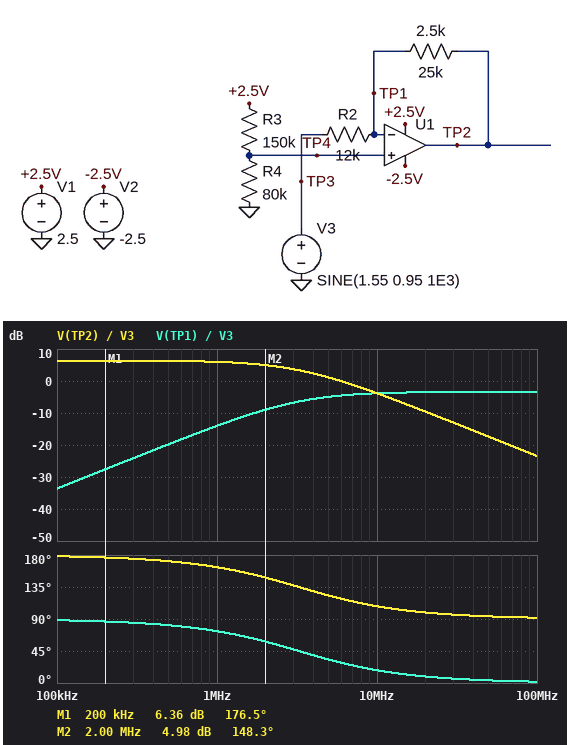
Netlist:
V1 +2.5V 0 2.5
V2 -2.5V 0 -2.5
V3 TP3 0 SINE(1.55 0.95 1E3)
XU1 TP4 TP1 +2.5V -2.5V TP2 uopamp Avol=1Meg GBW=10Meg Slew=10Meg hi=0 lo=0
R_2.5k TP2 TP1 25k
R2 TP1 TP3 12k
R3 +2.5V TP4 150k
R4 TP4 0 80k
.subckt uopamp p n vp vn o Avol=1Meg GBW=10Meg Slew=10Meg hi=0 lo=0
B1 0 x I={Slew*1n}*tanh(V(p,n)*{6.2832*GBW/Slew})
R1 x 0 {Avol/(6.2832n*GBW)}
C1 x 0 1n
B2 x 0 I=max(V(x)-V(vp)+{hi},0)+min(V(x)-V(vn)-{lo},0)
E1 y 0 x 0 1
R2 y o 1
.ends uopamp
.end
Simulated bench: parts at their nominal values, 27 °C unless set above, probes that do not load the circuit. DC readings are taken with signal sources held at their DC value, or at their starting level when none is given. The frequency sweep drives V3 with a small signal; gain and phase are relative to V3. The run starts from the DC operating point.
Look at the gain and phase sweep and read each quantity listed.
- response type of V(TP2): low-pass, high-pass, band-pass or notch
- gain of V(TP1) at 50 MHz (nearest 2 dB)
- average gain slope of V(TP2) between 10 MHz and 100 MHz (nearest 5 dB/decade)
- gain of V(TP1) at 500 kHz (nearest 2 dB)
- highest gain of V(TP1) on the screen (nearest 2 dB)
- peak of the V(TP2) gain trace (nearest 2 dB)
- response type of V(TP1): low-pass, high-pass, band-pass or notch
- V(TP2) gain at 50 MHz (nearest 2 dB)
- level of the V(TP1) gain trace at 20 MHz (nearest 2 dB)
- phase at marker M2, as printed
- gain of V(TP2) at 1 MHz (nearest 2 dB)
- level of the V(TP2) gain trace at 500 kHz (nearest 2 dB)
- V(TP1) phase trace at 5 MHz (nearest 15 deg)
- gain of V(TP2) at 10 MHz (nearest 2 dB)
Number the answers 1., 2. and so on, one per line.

1. low-pass
2. -4 dB
3. -20 dB/decade
4. -20 dB
5. -4 dB
6. 6 dB
7. high-pass
8. -18 dB
9. -4 dB
10. 148.3 deg
11. 6 dB
12. 6 dB
13. 30 deg
14. -4 dB
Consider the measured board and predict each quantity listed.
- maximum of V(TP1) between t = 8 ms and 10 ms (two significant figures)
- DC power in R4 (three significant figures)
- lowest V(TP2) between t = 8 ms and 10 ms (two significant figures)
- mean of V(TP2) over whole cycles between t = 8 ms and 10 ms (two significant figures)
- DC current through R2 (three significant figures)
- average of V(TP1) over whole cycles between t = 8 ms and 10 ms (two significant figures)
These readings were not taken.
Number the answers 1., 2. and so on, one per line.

1. 880 mV
2. 9.45 µW
3. -2.5 V
4. -550 mV
5. 56.7 µA
6. 870 mV
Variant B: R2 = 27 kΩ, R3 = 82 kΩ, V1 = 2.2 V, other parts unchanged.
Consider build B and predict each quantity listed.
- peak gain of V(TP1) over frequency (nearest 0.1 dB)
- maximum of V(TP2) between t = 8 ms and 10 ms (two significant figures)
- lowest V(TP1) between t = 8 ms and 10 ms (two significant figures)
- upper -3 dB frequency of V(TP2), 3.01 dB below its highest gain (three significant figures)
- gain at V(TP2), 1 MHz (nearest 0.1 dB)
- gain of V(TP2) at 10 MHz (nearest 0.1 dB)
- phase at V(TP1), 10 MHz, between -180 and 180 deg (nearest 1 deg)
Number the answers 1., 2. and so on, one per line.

1. -6.4 dB
2. 1.5 V
3. 1.1 V
4. 5.19 MHz
5. -0.8 dB
6. -7.4 dB
7. 27 deg
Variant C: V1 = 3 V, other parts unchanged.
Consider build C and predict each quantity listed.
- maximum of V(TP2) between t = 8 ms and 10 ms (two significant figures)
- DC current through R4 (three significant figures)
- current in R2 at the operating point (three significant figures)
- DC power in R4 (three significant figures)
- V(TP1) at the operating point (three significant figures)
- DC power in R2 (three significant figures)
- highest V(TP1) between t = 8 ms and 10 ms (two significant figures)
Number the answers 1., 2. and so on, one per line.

1. 2.0 V
2. 13.0 µA
3. 42.2 µA
4. 13.6 µW
5. 1.04 V
6. 21.4 µW
7. 1.0 V
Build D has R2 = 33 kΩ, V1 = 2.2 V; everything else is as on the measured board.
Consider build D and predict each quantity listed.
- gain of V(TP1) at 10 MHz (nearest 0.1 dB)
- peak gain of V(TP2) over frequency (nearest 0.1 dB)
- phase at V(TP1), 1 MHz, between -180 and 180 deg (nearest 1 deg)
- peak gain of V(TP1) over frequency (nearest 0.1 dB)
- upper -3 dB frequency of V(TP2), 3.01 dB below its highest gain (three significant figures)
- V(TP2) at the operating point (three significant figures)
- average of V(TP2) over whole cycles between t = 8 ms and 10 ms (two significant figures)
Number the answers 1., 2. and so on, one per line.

1. -8.5 dB
2. -2.4 dB
3. 80 deg
4. -7.3 dB
5. 5.69 MHz
6. 171 mV
7. 170 mV
